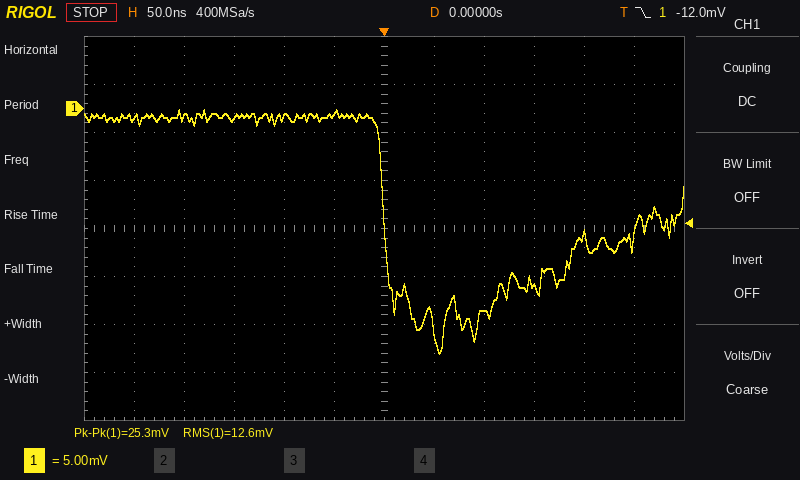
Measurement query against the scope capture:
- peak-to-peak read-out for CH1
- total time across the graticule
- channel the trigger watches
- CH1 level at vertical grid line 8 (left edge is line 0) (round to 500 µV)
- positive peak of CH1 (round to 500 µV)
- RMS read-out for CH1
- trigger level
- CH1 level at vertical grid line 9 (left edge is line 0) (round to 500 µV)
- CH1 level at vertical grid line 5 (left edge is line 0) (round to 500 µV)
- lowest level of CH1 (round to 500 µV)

25.3 mV
600 ns
CH1
-21.0 mV
0.0 mV
12.6 mV
-12.0 mV
-18.5 mV
-500 µV
-25.5 mV
